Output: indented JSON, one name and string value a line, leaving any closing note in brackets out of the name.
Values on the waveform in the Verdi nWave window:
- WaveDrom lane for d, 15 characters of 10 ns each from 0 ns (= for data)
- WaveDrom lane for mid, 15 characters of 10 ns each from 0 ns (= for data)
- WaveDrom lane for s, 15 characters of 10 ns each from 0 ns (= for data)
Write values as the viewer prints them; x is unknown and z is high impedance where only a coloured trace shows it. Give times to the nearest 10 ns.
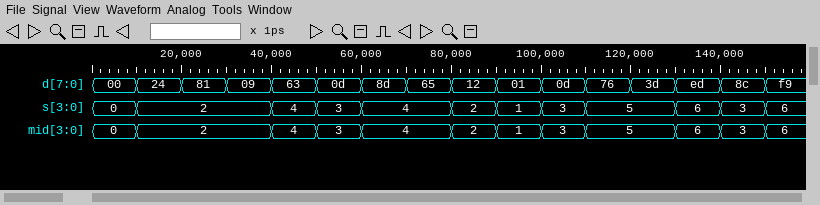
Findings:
{
  "WaveDrom lane for d, 15 characters of 10 ns each from 0 ns": "{name: 'd', wave: '===============', data: '00 24 81 09 63 0d 8d 65 12 01 0d 76 3d ed 8c'}",
  "WaveDrom lane for mid, 15 characters of 10 ns each from 0 ns": "{name: 'mid', wave: '==..===.====.==', data: '0 2 4 3 4 2 1 3 5 6 3'}",
  "WaveDrom lane for s, 15 characters of 10 ns each from 0 ns": "{name: 's', wave: '==..===.====.==', data: '0 2 4 3 4 2 1 3 5 6 3'}"
}
